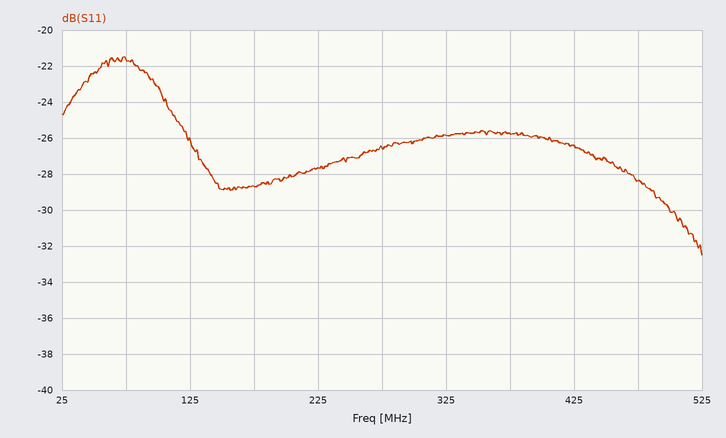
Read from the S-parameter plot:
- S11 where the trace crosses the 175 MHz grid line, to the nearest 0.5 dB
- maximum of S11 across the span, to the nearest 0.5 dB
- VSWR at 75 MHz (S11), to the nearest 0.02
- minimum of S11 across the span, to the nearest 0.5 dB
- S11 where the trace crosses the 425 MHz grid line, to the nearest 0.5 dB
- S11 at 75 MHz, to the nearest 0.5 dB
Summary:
-28.5 dB
-21.5 dB
1.18
-32.5 dB
-26.5 dB
-21.5 dB
